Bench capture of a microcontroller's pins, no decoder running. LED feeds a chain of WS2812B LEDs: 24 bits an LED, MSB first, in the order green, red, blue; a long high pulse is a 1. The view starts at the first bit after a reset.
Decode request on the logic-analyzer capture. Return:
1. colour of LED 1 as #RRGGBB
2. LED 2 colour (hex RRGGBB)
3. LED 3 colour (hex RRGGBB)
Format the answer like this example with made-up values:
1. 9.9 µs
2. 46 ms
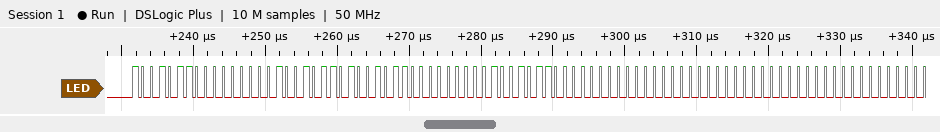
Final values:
1. #009696
2. #009696
3. #000000
